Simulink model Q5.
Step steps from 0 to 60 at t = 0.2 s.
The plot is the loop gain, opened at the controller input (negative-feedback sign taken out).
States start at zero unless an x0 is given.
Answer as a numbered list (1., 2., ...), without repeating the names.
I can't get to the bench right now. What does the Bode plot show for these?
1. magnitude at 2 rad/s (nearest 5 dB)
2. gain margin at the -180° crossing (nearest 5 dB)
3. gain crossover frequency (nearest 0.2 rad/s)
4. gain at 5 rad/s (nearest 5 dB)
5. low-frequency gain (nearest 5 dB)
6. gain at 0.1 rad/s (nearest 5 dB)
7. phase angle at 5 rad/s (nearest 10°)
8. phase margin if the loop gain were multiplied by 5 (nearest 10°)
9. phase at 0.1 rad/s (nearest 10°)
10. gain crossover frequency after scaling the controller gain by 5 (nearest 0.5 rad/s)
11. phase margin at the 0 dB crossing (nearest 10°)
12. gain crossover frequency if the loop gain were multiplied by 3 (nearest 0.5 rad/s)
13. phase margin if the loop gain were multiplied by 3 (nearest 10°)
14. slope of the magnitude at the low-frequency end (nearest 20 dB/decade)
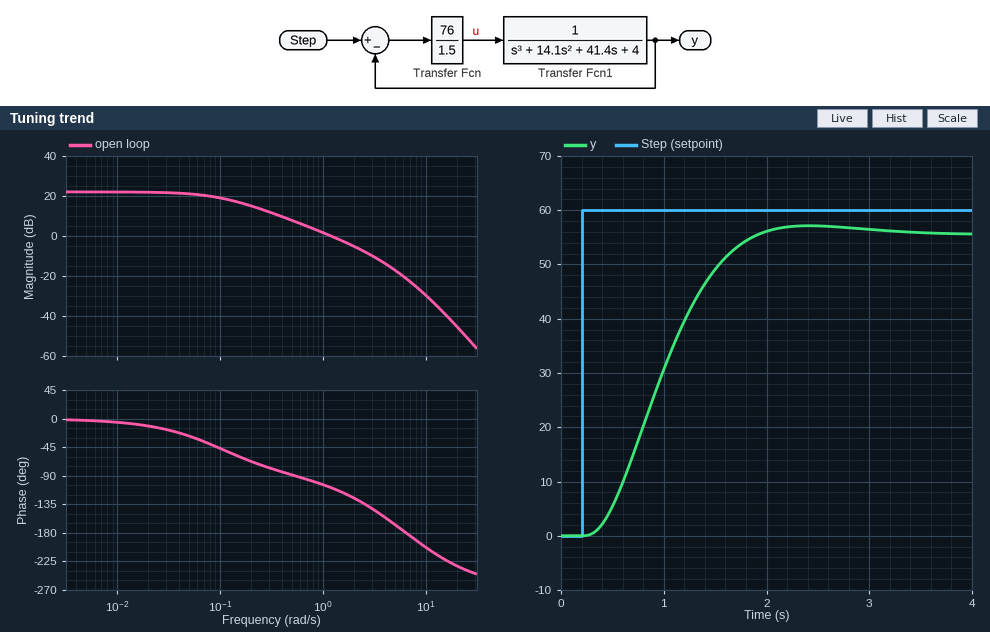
1. -5 dB
2. 20 dB
3. 1.2 rad/s
4. -15 dB
5. 20 dB
6. 20 dB
7. -170°
8. 20°
9. -50°
10. 4.0 rad/s
11. 70°
12. 3.0 rad/s
13. 40°
14. 0 dB/decade
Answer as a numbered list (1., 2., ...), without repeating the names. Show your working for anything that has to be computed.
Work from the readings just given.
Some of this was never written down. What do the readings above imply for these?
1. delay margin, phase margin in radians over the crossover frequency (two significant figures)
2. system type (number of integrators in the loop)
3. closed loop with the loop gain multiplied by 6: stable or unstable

1. 70 × π / 180 / 1.2 = 1.0 s
2. 0
3. stable
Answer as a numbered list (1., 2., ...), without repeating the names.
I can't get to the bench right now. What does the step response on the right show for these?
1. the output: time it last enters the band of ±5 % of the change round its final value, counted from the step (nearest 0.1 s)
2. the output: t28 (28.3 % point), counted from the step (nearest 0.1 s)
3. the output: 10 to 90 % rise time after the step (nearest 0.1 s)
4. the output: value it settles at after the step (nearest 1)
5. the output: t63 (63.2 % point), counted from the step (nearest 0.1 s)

1. 1.5 s
2. 0.5 s
3. 1.0 s
4. 56
5. 0.9 s
